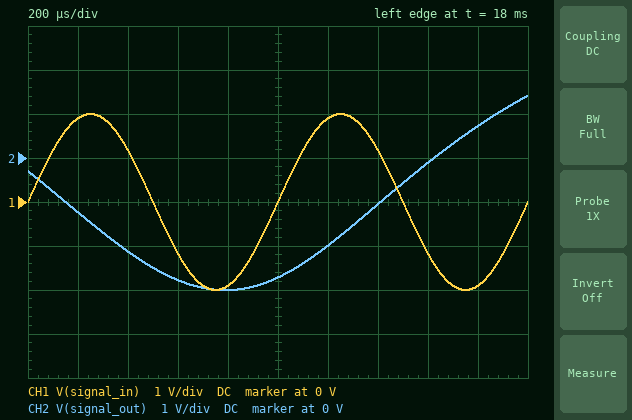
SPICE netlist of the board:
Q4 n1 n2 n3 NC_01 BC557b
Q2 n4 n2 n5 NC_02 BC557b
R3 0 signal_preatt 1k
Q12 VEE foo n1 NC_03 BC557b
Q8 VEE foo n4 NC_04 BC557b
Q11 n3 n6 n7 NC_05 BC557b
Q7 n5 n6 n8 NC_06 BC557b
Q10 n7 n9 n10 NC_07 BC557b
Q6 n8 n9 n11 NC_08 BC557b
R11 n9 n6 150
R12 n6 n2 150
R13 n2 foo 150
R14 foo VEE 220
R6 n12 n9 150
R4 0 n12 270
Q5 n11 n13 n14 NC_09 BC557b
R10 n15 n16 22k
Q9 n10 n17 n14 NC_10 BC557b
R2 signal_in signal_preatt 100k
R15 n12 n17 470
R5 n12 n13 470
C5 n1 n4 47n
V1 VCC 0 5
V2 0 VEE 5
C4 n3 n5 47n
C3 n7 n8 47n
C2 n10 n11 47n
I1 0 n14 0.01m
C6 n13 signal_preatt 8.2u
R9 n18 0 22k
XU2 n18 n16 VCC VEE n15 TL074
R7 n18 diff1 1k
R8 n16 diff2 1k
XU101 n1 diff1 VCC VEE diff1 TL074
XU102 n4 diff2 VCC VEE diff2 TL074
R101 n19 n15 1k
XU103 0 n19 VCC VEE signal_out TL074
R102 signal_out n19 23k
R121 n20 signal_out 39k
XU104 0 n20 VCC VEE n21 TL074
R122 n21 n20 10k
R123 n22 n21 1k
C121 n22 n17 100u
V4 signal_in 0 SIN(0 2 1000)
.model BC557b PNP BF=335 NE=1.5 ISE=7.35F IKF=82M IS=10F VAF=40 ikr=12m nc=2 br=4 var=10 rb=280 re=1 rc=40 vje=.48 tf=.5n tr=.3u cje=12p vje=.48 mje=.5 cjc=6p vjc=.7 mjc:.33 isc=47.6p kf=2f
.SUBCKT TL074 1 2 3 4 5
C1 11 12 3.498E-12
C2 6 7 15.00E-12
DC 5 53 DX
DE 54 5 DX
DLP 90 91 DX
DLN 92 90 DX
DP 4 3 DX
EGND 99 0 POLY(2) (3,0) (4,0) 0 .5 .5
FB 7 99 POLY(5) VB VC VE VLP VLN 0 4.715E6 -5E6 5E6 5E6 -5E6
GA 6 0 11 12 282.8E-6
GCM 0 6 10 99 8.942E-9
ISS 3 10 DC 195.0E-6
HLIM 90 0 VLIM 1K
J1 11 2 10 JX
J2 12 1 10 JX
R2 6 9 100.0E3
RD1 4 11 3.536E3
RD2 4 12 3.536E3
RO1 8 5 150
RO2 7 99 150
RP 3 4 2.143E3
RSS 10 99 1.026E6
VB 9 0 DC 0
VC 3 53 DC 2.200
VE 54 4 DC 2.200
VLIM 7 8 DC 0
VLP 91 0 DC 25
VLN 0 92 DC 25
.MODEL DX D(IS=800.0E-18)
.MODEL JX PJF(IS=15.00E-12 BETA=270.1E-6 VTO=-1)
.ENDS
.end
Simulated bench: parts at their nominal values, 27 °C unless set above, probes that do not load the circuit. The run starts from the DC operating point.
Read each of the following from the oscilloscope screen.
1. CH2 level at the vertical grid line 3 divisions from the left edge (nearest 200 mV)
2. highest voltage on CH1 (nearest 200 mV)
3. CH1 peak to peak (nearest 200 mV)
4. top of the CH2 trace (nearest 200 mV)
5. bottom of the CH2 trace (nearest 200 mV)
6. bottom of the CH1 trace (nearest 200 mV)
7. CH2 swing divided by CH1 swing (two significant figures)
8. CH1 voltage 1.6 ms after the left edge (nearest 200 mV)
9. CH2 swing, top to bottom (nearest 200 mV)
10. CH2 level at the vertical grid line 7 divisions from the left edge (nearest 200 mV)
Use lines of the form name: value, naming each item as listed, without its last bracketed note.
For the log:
CH2 level at the vertical grid line 3 divisions from the left edge: -2.8 V
highest voltage on CH1: 2.0 V
CH1 peak to peak: 4.0 V
top of the CH2 trace: 1.4 V
bottom of the CH2 trace: -3.0 V
bottom of the CH1 trace: -2.0 V
CH2 swing divided by CH1 swing: 1.1
CH1 voltage 1.6 ms after the left edge: -1.2 V
CH2 swing, top to bottom: 4.4 V
CH2 level at the vertical grid line 7 divisions from the left edge: -1.0 V
